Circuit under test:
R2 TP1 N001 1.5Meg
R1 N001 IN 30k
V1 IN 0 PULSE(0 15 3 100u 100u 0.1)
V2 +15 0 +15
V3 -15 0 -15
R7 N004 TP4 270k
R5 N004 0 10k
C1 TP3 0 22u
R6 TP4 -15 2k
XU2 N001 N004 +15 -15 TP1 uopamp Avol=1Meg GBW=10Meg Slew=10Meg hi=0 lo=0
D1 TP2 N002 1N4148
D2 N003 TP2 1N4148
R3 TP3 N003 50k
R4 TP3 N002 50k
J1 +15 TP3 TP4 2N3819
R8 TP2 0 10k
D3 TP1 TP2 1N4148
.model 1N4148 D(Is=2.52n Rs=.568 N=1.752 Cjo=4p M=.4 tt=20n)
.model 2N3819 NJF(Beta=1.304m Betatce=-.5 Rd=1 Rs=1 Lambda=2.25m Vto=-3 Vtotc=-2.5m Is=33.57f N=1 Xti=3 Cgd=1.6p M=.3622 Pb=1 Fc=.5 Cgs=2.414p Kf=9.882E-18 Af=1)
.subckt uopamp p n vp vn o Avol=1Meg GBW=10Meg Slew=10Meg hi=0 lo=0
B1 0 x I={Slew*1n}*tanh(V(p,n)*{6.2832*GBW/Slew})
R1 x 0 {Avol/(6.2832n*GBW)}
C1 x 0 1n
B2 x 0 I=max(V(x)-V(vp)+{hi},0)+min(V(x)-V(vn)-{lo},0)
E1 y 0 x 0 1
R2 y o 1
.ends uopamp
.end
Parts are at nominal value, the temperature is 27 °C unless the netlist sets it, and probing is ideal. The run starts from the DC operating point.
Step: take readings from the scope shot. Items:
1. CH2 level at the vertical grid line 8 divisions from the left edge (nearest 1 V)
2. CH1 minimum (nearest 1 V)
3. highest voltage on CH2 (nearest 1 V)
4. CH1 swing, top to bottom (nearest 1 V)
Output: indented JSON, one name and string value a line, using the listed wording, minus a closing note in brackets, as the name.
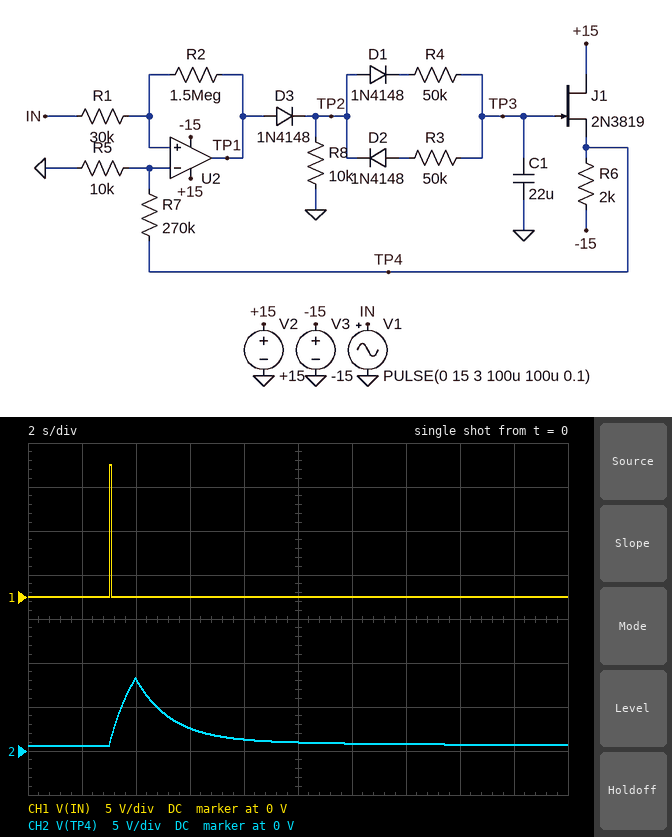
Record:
{
  "CH2 level at the vertical grid line 8 divisions from the left edge": "1 V",
  "CH1 minimum": "0 V",
  "highest voltage on CH2": "8 V",
  "CH1 swing, top to bottom": "15 V"
}
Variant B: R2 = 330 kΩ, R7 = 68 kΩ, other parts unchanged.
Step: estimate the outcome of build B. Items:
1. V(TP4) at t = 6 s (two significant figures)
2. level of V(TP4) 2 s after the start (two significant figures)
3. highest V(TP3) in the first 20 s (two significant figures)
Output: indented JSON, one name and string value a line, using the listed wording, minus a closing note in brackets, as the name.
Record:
{
  "V(TP4) at t = 6 s": "3.5 V",
  "level of V(TP4) 2 s after the start": "590 mV",
  "highest V(TP3) in the first 20 s": "9.8 V"
}
